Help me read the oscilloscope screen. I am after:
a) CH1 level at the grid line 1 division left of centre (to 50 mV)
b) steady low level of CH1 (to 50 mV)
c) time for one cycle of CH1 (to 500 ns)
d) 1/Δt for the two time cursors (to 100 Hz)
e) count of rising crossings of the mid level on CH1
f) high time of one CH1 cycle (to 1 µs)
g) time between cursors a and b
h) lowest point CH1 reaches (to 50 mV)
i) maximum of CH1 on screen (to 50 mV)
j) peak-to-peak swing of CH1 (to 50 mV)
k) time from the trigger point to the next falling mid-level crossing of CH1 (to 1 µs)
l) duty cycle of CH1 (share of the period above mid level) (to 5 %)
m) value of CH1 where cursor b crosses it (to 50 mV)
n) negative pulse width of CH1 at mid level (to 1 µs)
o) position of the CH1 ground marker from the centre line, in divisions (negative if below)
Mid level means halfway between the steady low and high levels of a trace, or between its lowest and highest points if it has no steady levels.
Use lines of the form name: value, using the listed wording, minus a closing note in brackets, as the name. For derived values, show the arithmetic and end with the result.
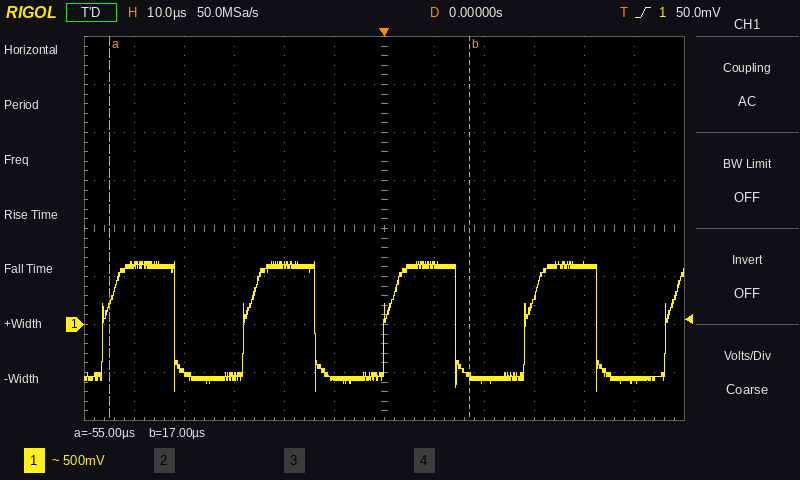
CH1 level at the grid line 1 division left of centre: -550 mV
steady low level of CH1: -550 mV
time for one cycle of CH1: 28.0 µs
1/Δt for the two time cursors: 1 / 72 µs ≈ 13.9 kHz
count of rising crossings of the mid level on CH1: 5
high time of one CH1 cycle: 14 µs
time between cursors a and b: 17 µs − (-55 µs) = 72 µs
lowest point CH1 reaches: -700 mV
maximum of CH1 on screen: 650 mV
peak-to-peak swing of CH1: 650 mV − (-700 mV) = 1.35 V
time from the trigger point to the next falling mid-level crossing of CH1: 14 µs
duty cycle of CH1 (share of the period above mid level): 14 µs / 28.0 µs ≈ 50 %
value of CH1 where cursor b crosses it: -550 mV
negative pulse width of CH1 at mid level: 14 µs
position of the CH1 ground marker from the centre line, in divisions: -2.0 div
